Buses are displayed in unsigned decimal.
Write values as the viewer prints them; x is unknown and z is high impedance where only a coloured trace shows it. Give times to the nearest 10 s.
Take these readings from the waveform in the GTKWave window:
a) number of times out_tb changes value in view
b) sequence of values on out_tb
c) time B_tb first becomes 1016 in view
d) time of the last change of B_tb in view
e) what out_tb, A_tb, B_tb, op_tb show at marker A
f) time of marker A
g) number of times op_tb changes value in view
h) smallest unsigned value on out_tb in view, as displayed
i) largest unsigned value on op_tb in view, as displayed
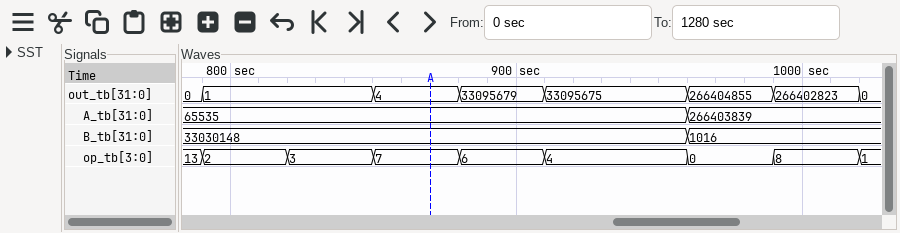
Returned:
7
0, 1, 4, 33095679, 33095675, 266404855, 266402823, 0
960 s
960 s
out_tb=4, A_tb=65535, B_tb=33030148, op_tb=7
870 s
8
0
13
